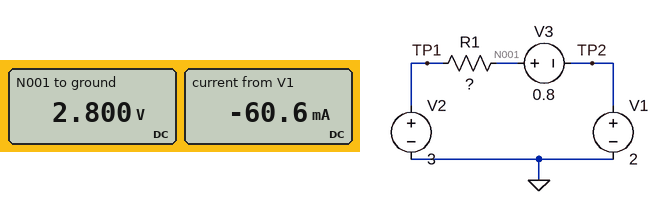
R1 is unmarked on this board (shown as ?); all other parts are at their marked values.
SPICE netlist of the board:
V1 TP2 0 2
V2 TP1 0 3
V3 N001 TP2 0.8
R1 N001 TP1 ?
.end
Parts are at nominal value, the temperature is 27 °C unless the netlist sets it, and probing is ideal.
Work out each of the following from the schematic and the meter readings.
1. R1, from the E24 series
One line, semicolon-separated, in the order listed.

3.3 Ω
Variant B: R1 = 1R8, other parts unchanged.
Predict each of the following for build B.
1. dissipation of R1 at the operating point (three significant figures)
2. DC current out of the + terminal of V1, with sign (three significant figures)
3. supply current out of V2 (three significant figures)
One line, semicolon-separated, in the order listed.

22.2 mW; -111 mA; 111 mA
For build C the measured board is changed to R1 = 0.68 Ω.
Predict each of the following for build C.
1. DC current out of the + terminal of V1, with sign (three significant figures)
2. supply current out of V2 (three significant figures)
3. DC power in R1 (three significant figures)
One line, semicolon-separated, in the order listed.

-294 mA; 294 mA; 58.8 mW
